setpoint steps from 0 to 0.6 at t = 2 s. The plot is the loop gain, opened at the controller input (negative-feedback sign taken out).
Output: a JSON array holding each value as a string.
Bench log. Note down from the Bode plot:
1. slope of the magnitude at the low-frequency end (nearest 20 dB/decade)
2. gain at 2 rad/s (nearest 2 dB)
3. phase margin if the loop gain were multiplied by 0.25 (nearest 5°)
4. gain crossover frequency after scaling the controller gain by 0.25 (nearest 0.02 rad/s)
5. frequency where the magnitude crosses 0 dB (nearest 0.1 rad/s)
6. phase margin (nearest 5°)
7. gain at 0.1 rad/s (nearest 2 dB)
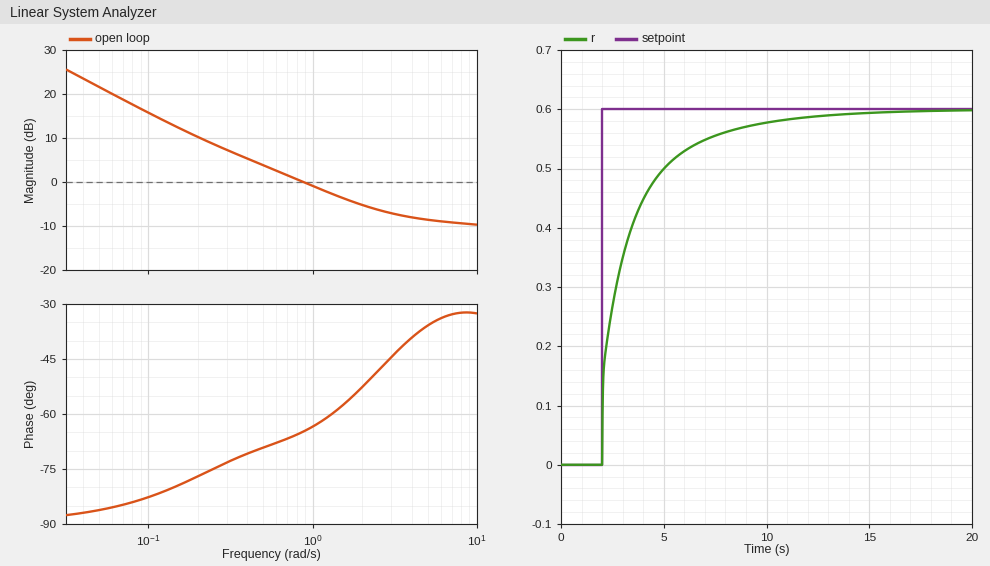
["-20 dB/decade", "-6 dB", "100°", "0.16 rad/s", "0.9 rad/s", "115°", "16 dB"]
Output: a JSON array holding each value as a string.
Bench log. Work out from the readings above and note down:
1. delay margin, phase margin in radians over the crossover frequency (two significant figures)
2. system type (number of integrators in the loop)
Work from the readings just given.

["2.2 s", "1"]
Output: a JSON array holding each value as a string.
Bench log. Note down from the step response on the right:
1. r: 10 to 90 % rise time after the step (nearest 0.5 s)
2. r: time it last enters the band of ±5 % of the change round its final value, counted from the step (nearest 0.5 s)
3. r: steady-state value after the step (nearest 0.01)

["4.5 s", "7.0 s", "0.60"]
